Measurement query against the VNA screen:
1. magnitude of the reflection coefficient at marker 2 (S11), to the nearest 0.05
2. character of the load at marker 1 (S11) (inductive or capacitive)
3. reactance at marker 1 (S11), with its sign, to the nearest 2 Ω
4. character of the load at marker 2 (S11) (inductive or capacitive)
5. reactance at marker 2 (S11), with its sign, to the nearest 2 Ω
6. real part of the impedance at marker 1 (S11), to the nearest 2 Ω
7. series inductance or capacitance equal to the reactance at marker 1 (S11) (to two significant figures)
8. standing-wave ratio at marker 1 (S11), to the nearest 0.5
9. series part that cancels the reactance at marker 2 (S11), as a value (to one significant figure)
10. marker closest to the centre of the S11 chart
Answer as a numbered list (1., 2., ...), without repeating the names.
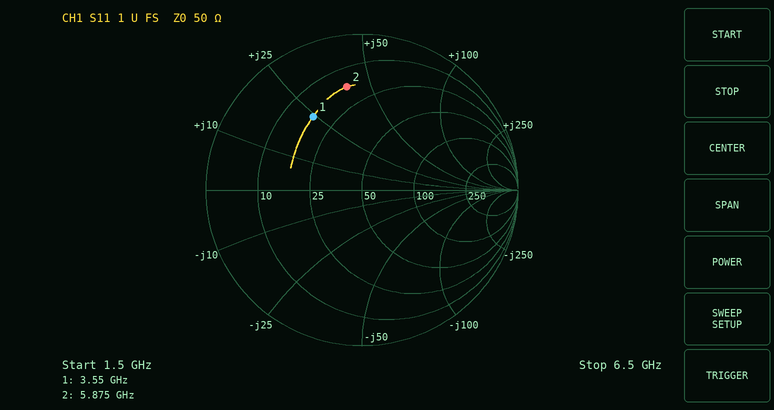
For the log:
1. 0.65
2. inductive
3. +24 Ω
4. inductive
5. +40 Ω
6. 18 Ω
7. 1.1 nH
8. 3.5
9. 700 fF
10. marker 1
